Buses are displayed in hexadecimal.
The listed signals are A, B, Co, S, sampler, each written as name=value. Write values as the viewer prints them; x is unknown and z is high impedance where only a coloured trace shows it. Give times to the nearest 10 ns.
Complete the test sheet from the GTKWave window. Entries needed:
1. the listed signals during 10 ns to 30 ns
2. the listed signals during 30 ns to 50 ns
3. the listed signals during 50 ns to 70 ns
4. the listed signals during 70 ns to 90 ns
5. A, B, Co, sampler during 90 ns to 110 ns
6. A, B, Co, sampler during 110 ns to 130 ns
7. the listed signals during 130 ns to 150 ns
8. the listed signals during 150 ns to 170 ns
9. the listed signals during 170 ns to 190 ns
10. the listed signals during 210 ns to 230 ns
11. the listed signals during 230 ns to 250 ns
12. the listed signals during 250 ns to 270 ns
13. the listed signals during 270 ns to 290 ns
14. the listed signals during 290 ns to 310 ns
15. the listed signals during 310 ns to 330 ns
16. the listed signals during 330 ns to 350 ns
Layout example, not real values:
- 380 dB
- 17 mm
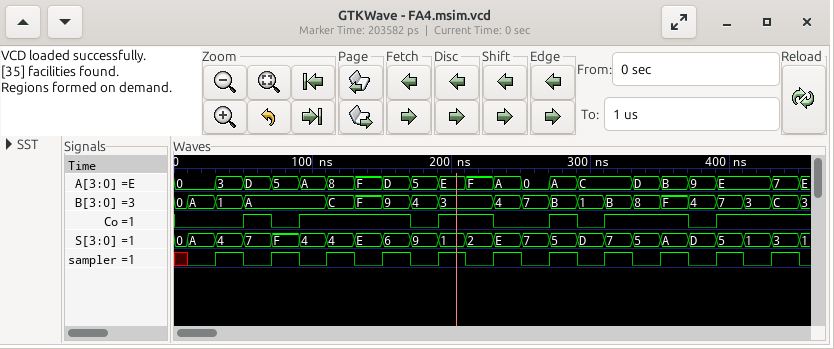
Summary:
- A=0, B=A, Co=0, S=A, sampler=0
- A=3, B=1, Co=0, S=4, sampler=1
- A=D, B=A, Co=1, S=7, sampler=0
- A=5, B=A, Co=0, S=F, sampler=1
- A=A, B=A, Co=1, sampler=0
- A=8, B=C, Co=1, sampler=1
- A=F, B=F, Co=1, S=E, sampler=0
- A=D, B=9, Co=1, S=6, sampler=1
- A=5, B=4, Co=0, S=9, sampler=0
- A=F, B=3, Co=1, S=2, sampler=0
- A=A, B=4, Co=0, S=E, sampler=1
- A=0, B=7, Co=0, S=7, sampler=0
- A=A, B=B, Co=1, S=5, sampler=1
- A=C, B=1, Co=0, S=D, sampler=0
- A=C, B=B, Co=1, S=7, sampler=1
- A=D, B=8, Co=1, S=5, sampler=0
